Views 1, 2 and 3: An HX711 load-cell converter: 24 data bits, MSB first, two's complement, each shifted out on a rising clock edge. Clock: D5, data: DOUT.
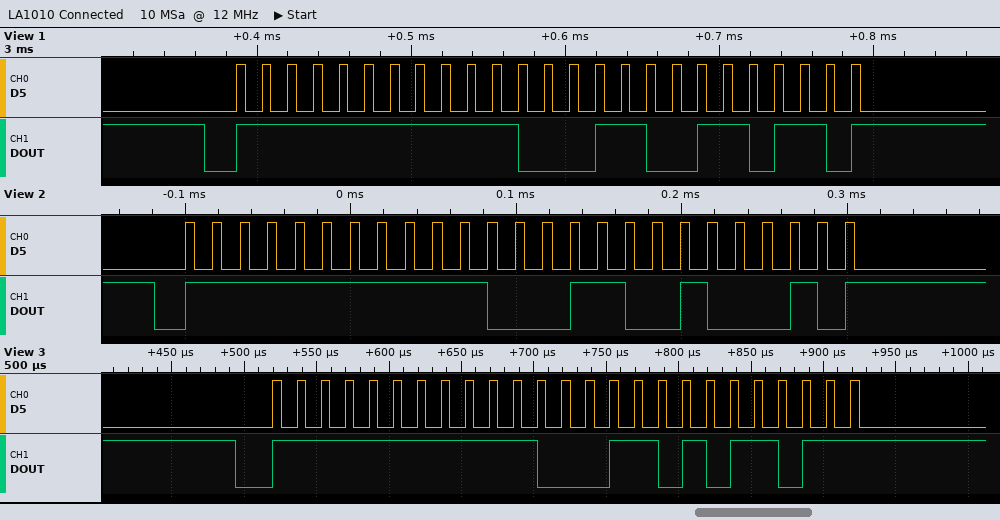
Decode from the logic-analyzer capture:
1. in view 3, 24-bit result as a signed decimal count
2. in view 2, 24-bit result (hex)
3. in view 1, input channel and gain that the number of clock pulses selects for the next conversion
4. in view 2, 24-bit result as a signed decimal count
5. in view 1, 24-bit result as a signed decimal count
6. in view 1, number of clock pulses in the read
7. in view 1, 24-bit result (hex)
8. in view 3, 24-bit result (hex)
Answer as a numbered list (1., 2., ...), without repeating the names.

1. -7333
2. 0xFFE322
3. channel A, gain 128
4. -7390
5. -7370
6. 25
7. 0xFFE336
8. 0xFFE35B
